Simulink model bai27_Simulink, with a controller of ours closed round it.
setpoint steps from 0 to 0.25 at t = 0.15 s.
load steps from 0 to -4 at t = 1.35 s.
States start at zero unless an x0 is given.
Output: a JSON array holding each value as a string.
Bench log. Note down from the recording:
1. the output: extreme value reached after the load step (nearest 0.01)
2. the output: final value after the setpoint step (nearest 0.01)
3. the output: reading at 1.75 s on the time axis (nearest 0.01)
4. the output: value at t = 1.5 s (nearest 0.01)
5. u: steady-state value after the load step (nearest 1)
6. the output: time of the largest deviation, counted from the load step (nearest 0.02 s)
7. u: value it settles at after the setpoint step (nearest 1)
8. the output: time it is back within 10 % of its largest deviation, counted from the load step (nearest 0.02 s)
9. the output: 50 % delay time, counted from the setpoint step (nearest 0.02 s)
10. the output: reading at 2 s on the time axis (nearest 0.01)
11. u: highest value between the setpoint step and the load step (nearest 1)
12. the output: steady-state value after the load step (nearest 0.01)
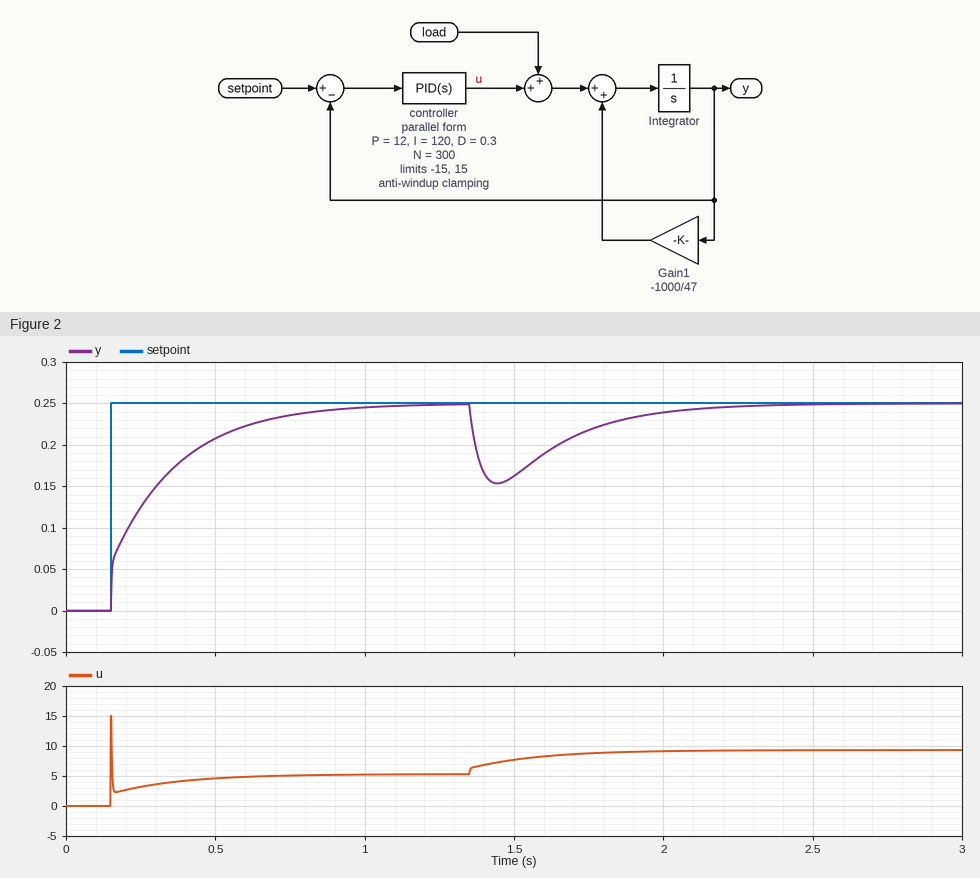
["0.15", "0.25", "0.22", "0.16", "9", "0.10 s", "5", "0.68 s", "0.10 s", "0.24", "15", "0.25"]
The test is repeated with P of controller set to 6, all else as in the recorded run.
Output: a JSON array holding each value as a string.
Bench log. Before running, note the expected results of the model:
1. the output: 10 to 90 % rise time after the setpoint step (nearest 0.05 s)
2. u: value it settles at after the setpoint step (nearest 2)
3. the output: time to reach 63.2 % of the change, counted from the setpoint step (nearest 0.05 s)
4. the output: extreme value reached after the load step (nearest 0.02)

["0.40 s", "6", "0.20 s", "0.14"]
